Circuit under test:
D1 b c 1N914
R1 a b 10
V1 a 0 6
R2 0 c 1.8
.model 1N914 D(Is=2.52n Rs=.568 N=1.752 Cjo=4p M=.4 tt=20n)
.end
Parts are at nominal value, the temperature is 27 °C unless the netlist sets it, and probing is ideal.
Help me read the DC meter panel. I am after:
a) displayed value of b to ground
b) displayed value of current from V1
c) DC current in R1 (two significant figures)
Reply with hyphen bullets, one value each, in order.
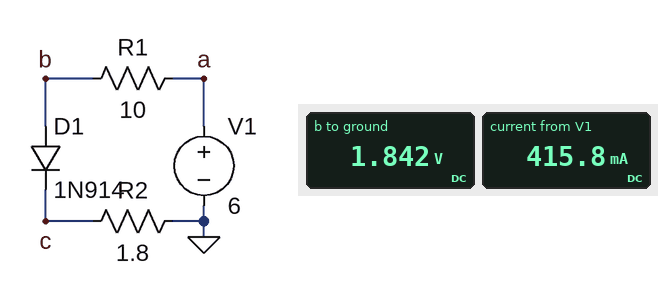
- 1.842 V
- 415.8 mA
- 420 mA
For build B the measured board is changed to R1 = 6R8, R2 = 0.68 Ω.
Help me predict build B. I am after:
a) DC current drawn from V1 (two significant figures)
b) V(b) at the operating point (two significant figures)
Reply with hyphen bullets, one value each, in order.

- 640 mA
- 1.7 V
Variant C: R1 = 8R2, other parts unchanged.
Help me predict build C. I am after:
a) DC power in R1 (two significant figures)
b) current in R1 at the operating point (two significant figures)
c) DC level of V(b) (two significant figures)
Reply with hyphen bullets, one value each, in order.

- 1.9 W
- 490 mA
- 2.0 V
